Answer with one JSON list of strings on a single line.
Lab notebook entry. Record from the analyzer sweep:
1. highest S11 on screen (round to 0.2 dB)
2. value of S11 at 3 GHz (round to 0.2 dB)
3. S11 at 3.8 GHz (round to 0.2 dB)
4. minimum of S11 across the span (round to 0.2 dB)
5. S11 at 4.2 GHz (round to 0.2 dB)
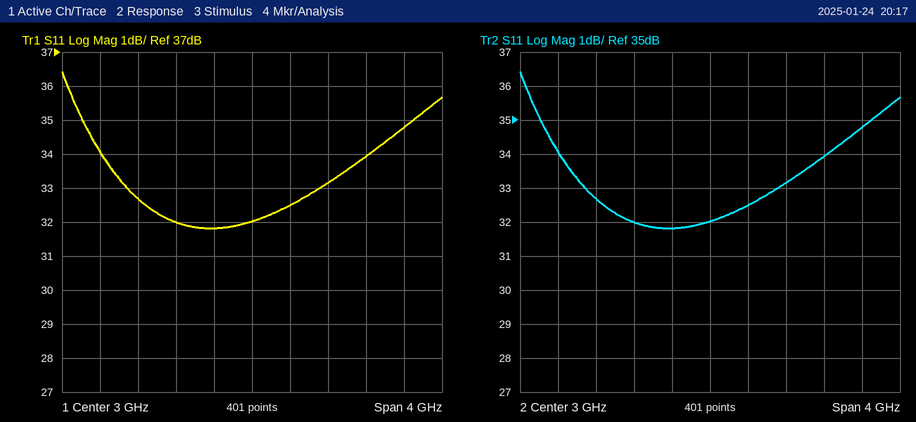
["36.4 dB", "32.0 dB", "33.2 dB", "31.8 dB", "34.0 dB"]
